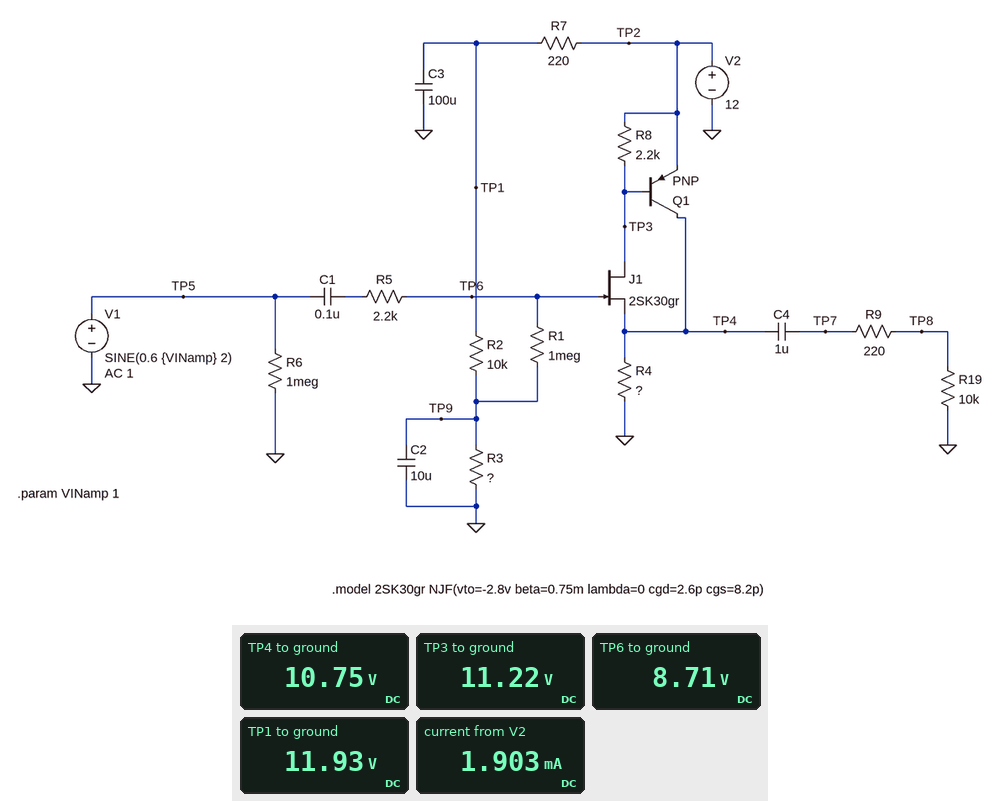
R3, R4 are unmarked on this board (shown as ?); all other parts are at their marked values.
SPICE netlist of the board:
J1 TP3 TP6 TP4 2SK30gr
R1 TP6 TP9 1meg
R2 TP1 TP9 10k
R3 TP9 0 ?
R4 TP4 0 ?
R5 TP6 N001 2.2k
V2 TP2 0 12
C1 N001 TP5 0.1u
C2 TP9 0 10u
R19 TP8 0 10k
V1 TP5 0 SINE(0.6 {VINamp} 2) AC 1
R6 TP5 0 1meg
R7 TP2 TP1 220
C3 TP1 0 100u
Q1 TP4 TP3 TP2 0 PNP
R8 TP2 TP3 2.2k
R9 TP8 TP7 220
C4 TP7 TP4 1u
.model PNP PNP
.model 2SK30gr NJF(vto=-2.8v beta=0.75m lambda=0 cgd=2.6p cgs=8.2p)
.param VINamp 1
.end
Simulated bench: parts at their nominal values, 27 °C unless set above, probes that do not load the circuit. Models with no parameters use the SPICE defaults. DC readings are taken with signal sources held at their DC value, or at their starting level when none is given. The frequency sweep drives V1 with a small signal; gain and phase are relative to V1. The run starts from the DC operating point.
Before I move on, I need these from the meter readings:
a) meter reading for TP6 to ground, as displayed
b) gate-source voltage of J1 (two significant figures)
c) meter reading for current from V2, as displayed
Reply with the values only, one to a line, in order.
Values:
8.71 V
-2.0 V
1.903 mA
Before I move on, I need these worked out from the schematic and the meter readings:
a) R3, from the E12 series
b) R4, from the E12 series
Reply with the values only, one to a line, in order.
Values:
27 kΩ
6.8 kΩ
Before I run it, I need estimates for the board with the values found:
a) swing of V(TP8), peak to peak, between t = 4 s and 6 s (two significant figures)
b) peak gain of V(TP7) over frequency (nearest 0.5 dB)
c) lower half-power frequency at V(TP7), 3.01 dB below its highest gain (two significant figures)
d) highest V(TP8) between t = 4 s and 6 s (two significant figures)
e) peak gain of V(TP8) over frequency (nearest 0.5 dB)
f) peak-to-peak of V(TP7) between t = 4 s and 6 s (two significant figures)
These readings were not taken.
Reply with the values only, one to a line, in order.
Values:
170 mV
-4.0 dB
16 Hz
87 mV
-4.5 dB
180 mV
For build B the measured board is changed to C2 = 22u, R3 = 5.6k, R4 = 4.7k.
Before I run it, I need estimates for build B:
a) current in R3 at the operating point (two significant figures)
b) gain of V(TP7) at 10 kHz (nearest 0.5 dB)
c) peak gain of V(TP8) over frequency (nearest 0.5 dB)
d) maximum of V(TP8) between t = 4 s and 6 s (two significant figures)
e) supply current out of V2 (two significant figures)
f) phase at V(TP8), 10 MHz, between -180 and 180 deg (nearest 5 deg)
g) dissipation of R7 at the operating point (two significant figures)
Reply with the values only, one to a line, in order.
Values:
760 µA
0 dB
3.0 dB
97 mV
2.1 mA
-10 deg
130 µW
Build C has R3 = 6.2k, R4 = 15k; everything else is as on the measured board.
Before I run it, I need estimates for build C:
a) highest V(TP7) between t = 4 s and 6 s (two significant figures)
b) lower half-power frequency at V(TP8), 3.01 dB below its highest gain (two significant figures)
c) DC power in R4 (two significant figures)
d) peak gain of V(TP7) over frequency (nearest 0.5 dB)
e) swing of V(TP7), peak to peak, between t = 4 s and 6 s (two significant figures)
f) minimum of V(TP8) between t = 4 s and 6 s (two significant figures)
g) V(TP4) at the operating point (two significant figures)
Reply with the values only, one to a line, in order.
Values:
99 mV
24 Hz
3.0 mW
1.5 dB
200 mV
-97 mV
6.7 V
